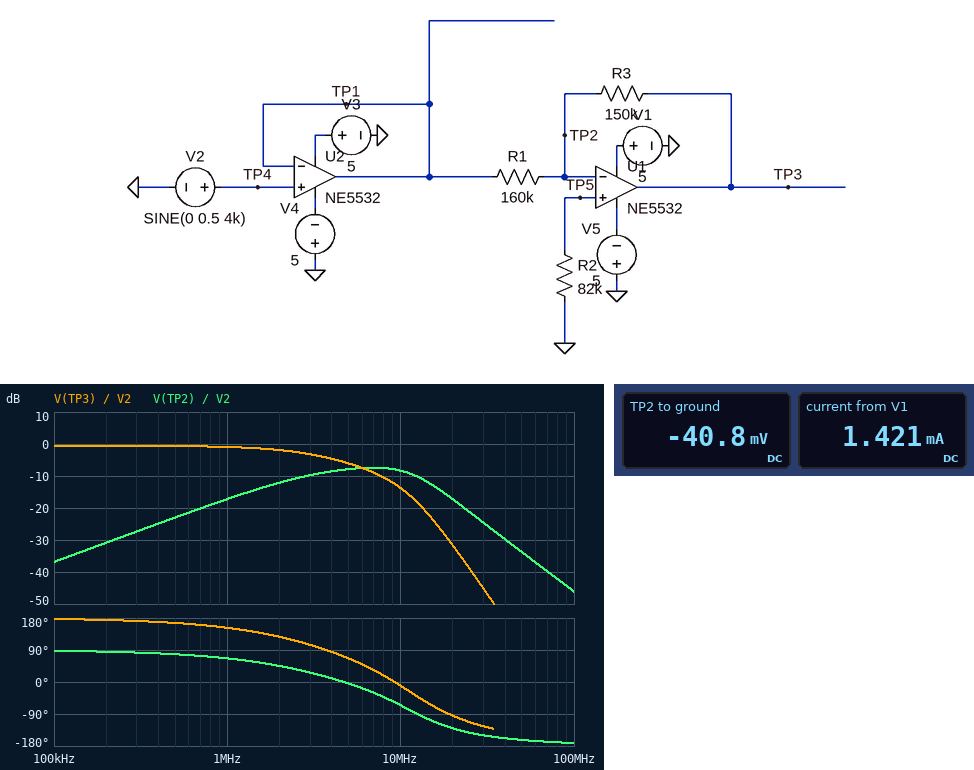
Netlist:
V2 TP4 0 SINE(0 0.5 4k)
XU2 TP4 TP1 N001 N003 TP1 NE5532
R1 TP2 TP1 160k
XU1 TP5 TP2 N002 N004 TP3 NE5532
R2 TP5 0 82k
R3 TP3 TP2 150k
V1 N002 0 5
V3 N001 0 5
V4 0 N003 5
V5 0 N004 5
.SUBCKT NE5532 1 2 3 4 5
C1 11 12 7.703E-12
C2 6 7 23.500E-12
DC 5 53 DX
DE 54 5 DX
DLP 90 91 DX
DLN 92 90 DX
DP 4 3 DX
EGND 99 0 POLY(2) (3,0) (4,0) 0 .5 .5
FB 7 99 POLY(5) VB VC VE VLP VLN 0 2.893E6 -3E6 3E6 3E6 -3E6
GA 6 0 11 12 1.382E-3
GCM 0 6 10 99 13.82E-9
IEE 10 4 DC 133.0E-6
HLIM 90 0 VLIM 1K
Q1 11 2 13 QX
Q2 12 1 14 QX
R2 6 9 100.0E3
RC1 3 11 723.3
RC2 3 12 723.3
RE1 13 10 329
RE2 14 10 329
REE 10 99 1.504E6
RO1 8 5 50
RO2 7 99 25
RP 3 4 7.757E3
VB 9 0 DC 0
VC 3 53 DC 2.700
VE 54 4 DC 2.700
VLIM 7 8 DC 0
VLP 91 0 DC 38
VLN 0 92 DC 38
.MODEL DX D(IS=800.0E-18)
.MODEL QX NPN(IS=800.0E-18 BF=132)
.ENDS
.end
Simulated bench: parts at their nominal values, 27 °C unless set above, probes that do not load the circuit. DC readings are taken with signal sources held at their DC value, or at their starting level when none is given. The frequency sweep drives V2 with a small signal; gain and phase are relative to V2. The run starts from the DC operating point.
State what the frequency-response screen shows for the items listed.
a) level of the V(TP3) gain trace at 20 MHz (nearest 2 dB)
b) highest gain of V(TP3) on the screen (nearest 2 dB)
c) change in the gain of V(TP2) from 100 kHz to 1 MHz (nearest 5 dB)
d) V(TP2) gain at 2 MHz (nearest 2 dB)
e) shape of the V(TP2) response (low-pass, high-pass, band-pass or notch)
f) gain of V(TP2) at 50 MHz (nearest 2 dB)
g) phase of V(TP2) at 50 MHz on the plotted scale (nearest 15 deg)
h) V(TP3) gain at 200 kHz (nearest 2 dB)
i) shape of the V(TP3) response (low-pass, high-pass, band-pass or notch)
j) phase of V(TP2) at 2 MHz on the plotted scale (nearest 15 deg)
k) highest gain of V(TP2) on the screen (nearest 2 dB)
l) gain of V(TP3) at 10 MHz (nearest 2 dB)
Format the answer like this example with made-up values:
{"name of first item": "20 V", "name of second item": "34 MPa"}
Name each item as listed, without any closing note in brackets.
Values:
{"level of the V(TP3) gain trace at 20 MHz": "-32 dB", "highest gain of V(TP3) on the screen": "0 dB", "change in the gain of V(TP2) from 100 kHz to 1 MHz": "20 dB", "V(TP2) gain at 2 MHz": "-12 dB", "shape of the V(TP2) response": "band-pass", "gain of V(TP2) at 50 MHz": "-34 dB", "phase of V(TP2) at 50 MHz on the plotted scale": "-165 deg", "V(TP3) gain at 200 kHz": "0 dB", "shape of the V(TP3) response": "low-pass", "phase of V(TP2) at 2 MHz on the plotted scale": "45 deg", "highest gain of V(TP2) on the screen": "-8 dB", "gain of V(TP3) at 10 MHz": "-14 dB"}
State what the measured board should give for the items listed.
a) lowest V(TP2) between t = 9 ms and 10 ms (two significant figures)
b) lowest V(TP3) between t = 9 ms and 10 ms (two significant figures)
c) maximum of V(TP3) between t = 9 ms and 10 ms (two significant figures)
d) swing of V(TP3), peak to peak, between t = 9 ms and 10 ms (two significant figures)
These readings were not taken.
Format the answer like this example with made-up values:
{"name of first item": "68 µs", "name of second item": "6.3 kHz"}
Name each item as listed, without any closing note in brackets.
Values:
{"lowest V(TP2) between t = 9 ms and 10 ms": "-41 mV", "lowest V(TP3) between t = 9 ms and 10 ms": "-470 mV", "maximum of V(TP3) between t = 9 ms and 10 ms": "460 mV", "swing of V(TP3), peak to peak, between t = 9 ms and 10 ms": "940 mV"}
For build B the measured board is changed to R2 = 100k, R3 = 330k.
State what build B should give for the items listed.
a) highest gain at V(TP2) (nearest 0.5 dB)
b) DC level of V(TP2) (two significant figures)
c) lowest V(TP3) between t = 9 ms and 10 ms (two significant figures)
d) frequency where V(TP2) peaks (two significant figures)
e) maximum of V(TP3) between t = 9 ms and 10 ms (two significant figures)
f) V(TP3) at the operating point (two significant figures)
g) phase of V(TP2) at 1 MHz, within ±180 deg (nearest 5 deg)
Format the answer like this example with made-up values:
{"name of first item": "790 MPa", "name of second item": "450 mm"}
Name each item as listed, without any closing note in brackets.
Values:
{"highest gain at V(TP2)": "-5.5 dB", "DC level of V(TP2)": "-50 mV", "lowest V(TP3) between t = 9 ms and 10 ms": "-1.0 V", "frequency where V(TP2) peaks": "6.2 MHz", "maximum of V(TP3) between t = 9 ms and 10 ms": "1.0 V", "V(TP3) at the operating point": "12 mV", "phase of V(TP2) at 1 MHz, within ±180 deg": "50 deg"}
